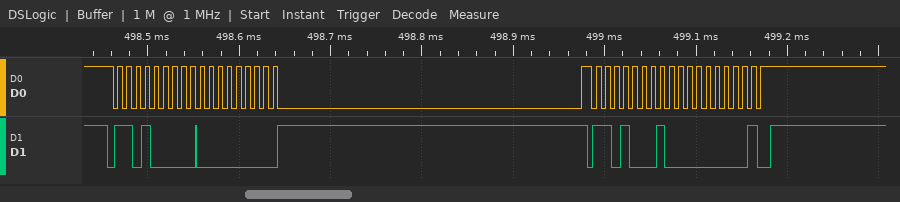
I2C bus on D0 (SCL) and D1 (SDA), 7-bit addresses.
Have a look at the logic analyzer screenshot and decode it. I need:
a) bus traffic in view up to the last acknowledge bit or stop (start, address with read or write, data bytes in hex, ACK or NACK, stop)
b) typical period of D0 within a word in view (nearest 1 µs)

start, address 68 write ACK, 00 ACK, repeated start, address 68 read ACK, 00 NACK, stop
10 µs
